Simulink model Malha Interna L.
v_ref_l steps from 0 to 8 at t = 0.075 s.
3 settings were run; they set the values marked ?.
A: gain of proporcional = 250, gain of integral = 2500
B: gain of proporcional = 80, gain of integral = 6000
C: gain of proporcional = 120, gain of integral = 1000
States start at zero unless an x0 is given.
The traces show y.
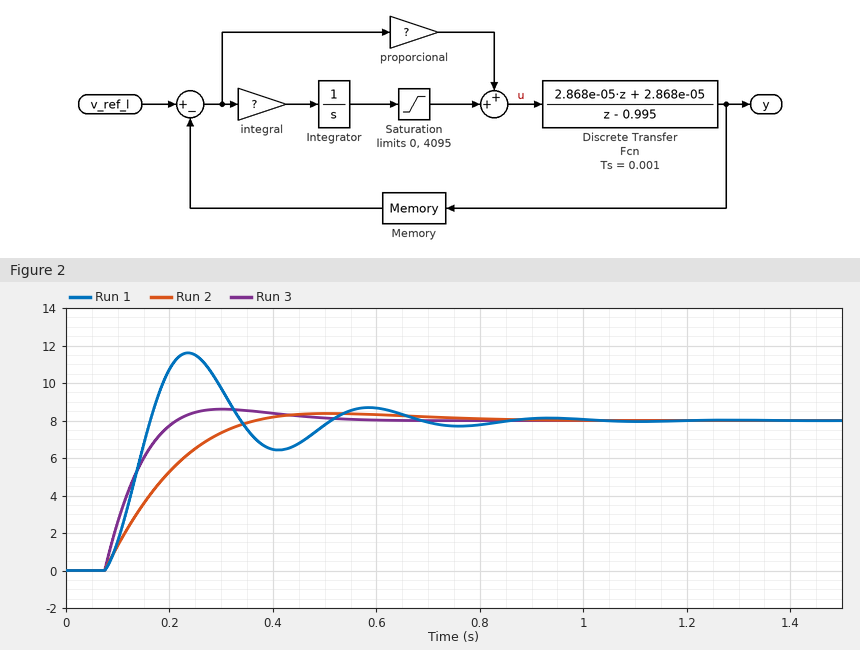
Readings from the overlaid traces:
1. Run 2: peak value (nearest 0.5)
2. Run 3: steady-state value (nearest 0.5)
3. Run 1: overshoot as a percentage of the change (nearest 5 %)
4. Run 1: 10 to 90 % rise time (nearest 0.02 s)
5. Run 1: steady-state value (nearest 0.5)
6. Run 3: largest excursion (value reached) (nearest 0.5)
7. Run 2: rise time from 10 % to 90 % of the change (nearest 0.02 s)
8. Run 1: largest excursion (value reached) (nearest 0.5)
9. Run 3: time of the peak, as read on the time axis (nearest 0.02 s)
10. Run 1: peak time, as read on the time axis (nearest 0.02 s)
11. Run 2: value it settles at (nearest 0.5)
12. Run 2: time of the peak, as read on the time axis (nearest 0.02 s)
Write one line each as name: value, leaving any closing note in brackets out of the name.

Run 2: peak value: 8.5
Run 3: steady-state value: 8.0
Run 1: overshoot as a percentage of the change: 45 %
Run 1: 10 to 90 % rise time: 0.06 s
Run 1: steady-state value: 8.0
Run 3: largest excursion (value reached): 8.5
Run 2: rise time from 10 % to 90 % of the change: 0.20 s
Run 1: largest excursion (value reached): 11.5
Run 3: time of the peak, as read on the time axis: 0.30 s
Run 1: peak time, as read on the time axis: 0.24 s
Run 2: value it settles at: 8.0
Run 2: time of the peak, as read on the time axis: 0.50 s
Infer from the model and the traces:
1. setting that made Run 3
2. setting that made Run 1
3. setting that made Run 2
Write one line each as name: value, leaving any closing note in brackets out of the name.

setting that made Run 3: A
setting that made Run 1: B
setting that made Run 2: C
